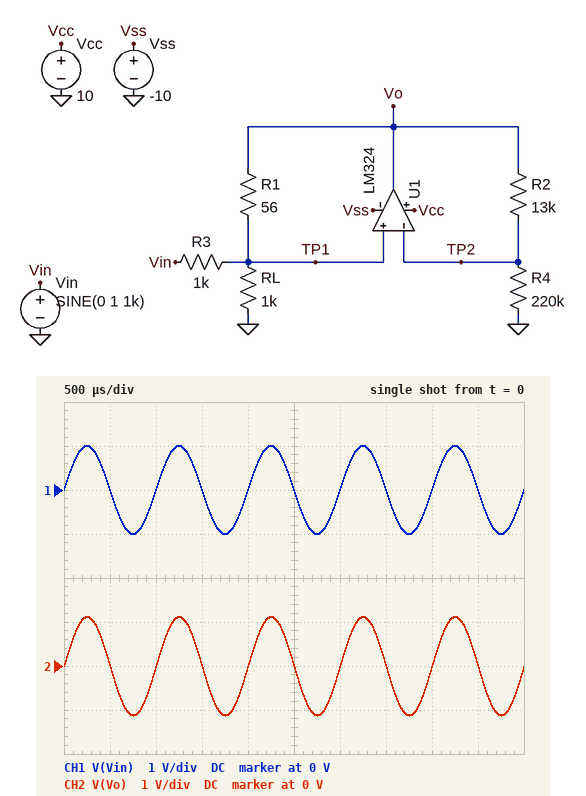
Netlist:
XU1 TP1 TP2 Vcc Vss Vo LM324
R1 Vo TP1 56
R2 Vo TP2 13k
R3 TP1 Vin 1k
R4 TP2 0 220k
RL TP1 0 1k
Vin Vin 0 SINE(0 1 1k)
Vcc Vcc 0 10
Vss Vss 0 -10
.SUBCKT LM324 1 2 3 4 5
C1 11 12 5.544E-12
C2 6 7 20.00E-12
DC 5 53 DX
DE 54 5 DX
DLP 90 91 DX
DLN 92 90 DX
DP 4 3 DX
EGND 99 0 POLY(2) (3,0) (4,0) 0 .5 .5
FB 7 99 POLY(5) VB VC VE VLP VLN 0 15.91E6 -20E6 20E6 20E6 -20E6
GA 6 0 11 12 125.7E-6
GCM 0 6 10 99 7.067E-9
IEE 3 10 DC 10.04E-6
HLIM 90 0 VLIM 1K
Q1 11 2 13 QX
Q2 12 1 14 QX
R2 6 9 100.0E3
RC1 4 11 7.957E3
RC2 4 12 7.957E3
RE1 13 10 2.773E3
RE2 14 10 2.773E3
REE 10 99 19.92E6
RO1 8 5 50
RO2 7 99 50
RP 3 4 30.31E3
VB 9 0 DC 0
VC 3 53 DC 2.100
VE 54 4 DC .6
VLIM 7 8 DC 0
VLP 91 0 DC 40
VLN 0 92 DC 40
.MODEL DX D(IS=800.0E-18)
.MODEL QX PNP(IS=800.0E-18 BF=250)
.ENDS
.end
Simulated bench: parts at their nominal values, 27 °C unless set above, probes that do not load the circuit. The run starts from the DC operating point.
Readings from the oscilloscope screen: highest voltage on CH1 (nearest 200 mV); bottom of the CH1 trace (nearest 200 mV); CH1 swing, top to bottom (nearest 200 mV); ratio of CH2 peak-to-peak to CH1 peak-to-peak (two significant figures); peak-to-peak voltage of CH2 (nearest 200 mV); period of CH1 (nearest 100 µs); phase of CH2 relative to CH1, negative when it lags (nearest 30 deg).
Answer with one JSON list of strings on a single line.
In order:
["1.0 V", "-1.0 V", "2.0 V", "1.1", "2.2 V", "1.0 ms", "0 deg"]
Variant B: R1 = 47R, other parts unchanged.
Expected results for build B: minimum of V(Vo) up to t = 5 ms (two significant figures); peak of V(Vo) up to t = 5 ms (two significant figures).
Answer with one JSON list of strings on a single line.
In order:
["-1.4 V", "1.4 V"]
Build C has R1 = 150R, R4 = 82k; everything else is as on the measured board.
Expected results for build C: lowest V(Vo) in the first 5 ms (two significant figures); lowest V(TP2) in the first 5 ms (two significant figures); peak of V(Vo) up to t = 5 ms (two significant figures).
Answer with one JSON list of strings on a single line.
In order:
["-1.2 V", "-1.1 V", "1.2 V"]
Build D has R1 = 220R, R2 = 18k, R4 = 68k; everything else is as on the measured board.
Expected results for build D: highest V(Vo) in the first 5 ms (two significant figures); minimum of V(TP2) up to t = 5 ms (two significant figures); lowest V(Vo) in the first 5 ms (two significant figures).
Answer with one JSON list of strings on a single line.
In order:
["1.6 V", "-1.3 V", "-1.6 V"]
